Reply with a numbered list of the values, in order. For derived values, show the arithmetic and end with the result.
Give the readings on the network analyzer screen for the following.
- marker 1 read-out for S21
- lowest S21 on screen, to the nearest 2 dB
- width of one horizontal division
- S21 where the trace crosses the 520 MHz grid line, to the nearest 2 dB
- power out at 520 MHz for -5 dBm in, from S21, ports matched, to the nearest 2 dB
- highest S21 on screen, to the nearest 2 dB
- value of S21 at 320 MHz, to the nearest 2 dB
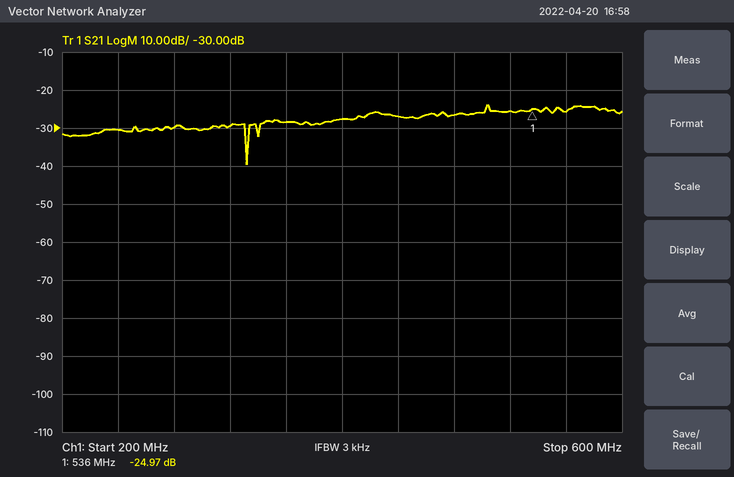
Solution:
1. -24.97 dB
2. -40 dB
3. 40 MHz
4. -26 dB
5. -5 dBm + (-26 dB) = -30 dBm
6. -24 dB
7. -30 dB
